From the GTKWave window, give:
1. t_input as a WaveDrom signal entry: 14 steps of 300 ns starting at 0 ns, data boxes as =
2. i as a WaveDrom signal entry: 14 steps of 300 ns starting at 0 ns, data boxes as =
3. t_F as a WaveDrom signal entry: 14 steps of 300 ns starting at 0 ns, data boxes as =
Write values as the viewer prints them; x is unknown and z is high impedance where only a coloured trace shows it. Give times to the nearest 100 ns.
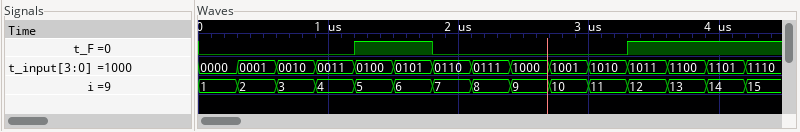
{name: 't_input', wave: '==============', data: '0000 0001 0010 0011 0100 0101 0110 0111 1000 1001 1010 1011 1100 1101'}
{name: 'i', wave: '==============', data: '1 2 3 4 5 6 7 8 9 10 11 12 13 14'}
{name: 't_F', wave: '0...1.0....1..'}
